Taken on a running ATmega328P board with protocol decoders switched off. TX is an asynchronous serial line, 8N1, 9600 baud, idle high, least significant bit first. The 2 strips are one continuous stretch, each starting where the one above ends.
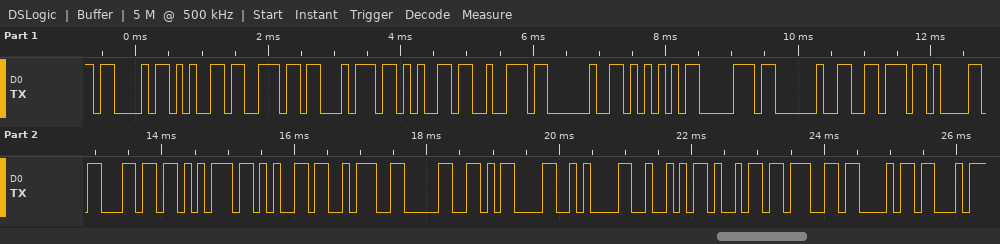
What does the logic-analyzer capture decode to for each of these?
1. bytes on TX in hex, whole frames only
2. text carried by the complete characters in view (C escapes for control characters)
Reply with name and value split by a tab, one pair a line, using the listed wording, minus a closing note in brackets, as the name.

bytes on TX in hex, whole frames only	43 65 6E 74 65 72 20 55 70 20 76 61 6C 75 65 3A 30 0D 0A 52 69 67 68
text carried by the complete characters in view	"Center Up value:0\r\nRigh"
